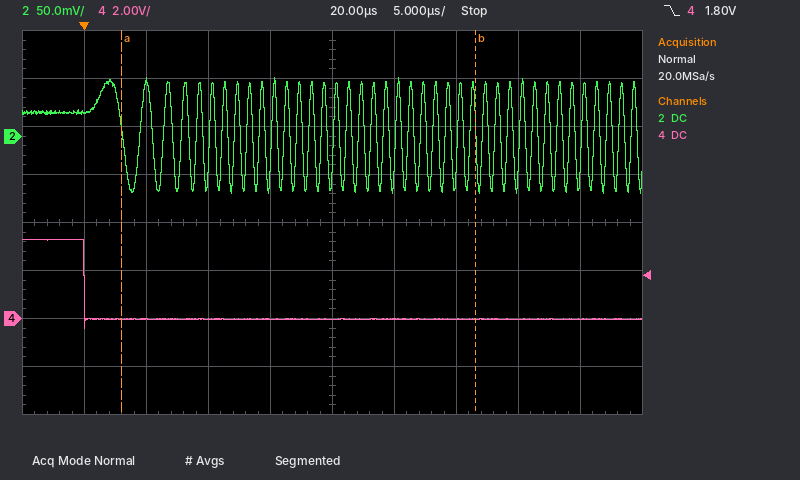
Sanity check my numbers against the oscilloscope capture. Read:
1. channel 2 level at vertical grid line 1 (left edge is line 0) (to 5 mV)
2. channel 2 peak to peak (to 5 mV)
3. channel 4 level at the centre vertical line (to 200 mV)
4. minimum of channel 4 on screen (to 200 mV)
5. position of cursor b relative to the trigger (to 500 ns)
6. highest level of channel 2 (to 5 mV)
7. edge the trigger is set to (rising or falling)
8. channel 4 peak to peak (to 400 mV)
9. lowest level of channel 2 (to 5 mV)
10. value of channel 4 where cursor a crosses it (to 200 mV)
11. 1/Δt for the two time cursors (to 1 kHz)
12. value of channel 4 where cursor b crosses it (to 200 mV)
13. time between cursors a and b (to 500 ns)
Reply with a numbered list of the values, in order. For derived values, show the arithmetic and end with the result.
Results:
1. 25 mV
2. 60 mV − (-60 mV) = 120 mV
3. 0.0 V
4. -400 mV
5. +31.5 µs
6. 60 mV
7. falling
8. 3.6 V
9. -60 mV
10. 0.0 V
11. 1 / 28.5 µs ≈ 35 kHz
12. 0.0 V
13. 28.5 µs
